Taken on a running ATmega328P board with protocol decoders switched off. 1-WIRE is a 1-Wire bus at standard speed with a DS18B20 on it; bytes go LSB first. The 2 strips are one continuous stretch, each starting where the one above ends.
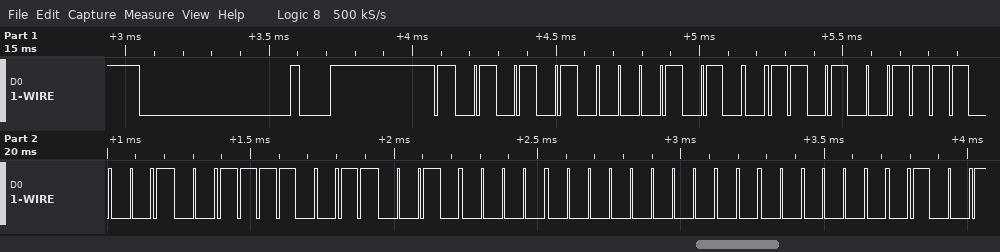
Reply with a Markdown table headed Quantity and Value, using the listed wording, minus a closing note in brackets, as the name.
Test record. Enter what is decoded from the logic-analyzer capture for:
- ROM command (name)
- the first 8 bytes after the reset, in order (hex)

| Quantity | Value |
|---|---|
| ROM command | Match ROM |
| the first 8 bytes after the reset, in order | 55 28 CB 23 CF 04 00 00 |
